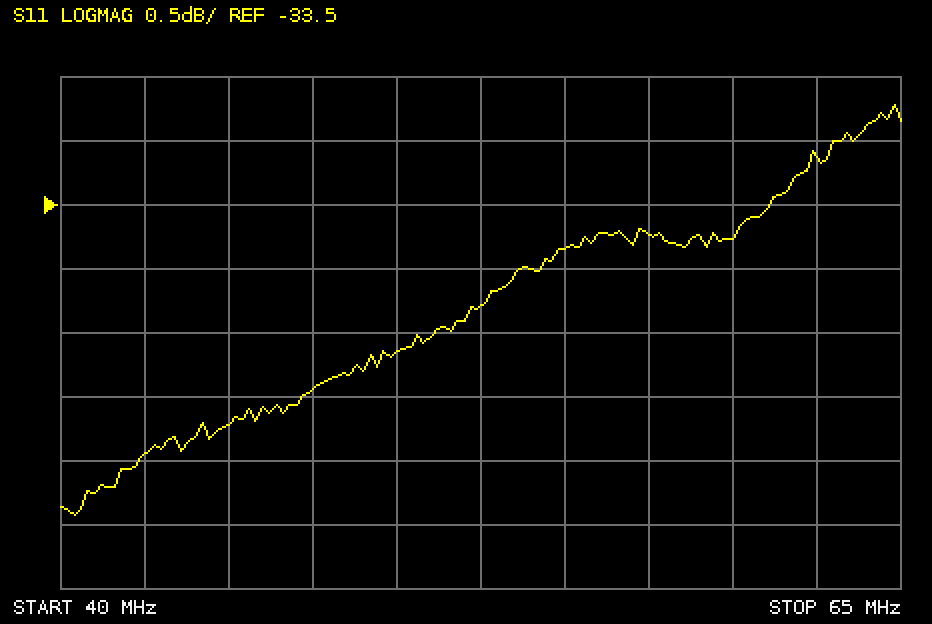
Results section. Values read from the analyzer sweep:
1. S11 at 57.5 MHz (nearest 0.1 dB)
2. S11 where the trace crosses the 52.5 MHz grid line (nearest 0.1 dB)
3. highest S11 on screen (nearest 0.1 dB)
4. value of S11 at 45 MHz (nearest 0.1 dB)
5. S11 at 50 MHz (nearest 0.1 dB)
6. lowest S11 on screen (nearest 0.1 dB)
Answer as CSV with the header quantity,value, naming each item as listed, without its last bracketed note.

quantity,value
S11 at 57.5 MHz,-33.7 dB
S11 where the trace crosses the 52.5 MHz grid line,-34.3 dB
highest S11 on screen,-32.7 dB
value of S11 at 45 MHz,-35.2 dB
S11 at 50 MHz,-34.6 dB
lowest S11 on screen,-35.9 dB
